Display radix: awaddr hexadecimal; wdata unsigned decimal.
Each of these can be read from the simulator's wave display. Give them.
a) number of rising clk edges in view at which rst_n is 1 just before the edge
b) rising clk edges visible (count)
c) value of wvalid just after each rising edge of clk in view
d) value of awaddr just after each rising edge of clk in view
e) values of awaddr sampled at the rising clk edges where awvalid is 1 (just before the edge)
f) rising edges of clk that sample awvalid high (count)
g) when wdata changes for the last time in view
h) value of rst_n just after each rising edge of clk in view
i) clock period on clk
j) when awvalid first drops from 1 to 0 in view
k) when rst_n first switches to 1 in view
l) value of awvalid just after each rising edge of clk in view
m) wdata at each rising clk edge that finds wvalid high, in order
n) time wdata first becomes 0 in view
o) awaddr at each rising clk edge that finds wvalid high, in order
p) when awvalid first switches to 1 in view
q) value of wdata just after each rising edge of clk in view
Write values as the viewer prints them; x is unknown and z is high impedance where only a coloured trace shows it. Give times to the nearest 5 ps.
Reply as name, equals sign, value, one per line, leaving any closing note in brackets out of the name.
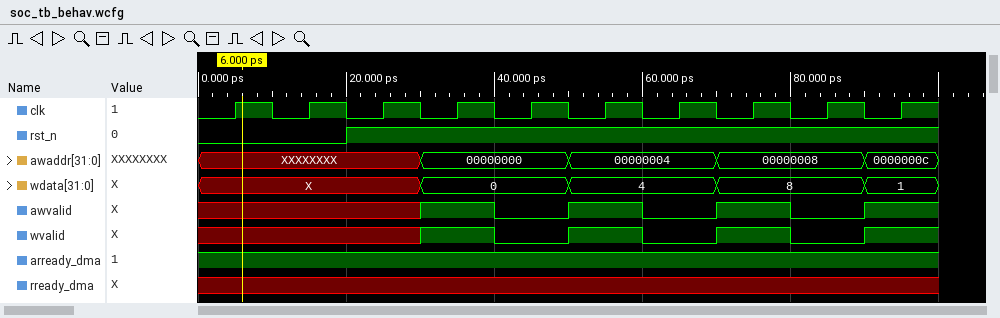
number of rising clk edges in view at which rst_n is 1 just before the edge = 8
rising clk edges visible = 10
value of wvalid just after each rising edge of clk in view = x x x 1 0 1 0 1 0 1
value of awaddr just after each rising edge of clk in view = XXXXXXXX, XXXXXXXX, XXXXXXXX, 00000000, 00000000, 00000004, 00000004, 00000008, 00000008, 0000000c
values of awaddr sampled at the rising clk edges where awvalid is 1 = 00000000, 00000004, 00000008, 0000000c
rising edges of clk that sample awvalid high = 4
when wdata changes for the last time in view = 90 ps
value of rst_n just after each rising edge of clk in view = 0 0 1 1 1 1 1 1 1 1
clock period on clk = 10 ps
when awvalid first drops from 1 to 0 in view = 40 ps
when rst_n first switches to 1 in view = 20 ps
value of awvalid just after each rising edge of clk in view = x x x 1 0 1 0 1 0 1
wdata at each rising clk edge that finds wvalid high, in order = 0, 4, 8, 1
time wdata first becomes 0 in view = 30 ps
awaddr at each rising clk edge that finds wvalid high, in order = 00000000, 00000004, 00000008, 0000000c
when awvalid first switches to 1 in view = 30 ps
value of wdata just after each rising edge of clk in view = X, X, X, 0, 0, 4, 4, 8, 8, 1
